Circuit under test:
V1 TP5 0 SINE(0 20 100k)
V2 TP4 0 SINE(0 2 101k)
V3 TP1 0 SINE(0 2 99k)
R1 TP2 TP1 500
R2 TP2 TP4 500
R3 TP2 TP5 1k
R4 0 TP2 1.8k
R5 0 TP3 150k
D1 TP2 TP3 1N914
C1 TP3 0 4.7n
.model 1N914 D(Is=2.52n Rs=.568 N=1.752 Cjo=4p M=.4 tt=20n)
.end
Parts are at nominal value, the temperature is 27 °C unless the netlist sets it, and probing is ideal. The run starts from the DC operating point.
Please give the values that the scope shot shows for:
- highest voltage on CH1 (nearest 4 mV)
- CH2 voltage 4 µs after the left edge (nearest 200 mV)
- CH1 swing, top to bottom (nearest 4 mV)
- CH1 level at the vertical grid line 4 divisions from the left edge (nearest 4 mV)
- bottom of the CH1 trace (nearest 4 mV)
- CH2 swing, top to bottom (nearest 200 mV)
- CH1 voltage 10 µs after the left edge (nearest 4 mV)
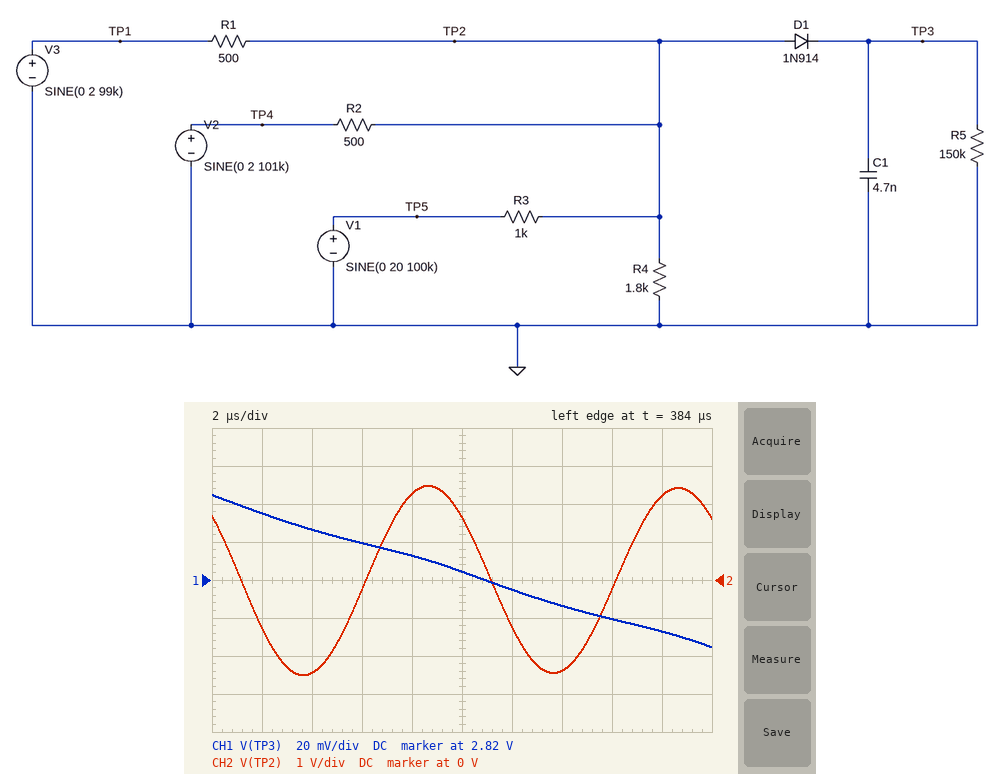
2.864 V
-2.4 V
80 mV
2.832 V
2.784 V
5.0 V
2.824 V
